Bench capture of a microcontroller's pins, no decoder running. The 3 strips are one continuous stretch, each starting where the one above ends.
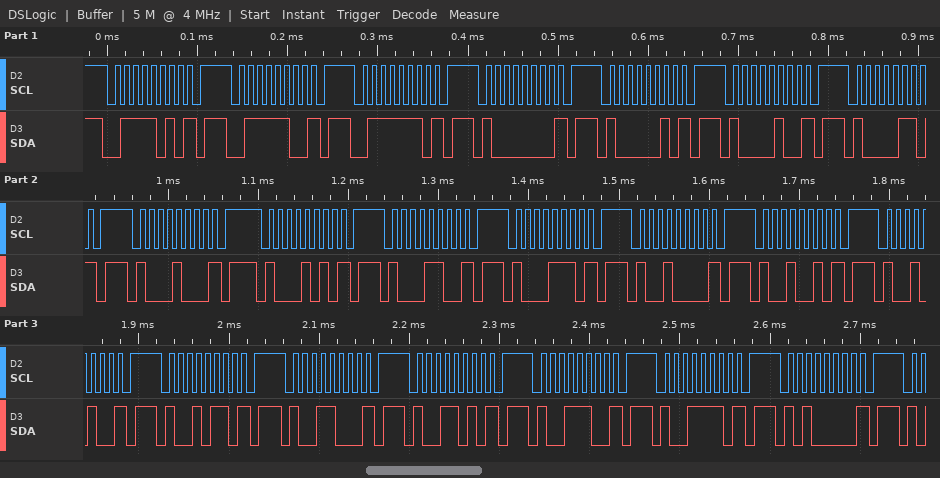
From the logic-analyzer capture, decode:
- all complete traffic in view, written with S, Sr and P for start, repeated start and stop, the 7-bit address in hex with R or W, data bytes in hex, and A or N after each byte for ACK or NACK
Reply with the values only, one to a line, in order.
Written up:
S 3DW N P S 3EW N P S 3FW N P S 40W N P S 41W N P S 42W N P S 43W N P S 44W N P S 45W N P S 46W N P S 47W N P S 48W N P S 49W N P S 4AW N P S 4BW N P S 4CW N P S 4DW N P S 4EW N P S 4FW N P S 50W N P
